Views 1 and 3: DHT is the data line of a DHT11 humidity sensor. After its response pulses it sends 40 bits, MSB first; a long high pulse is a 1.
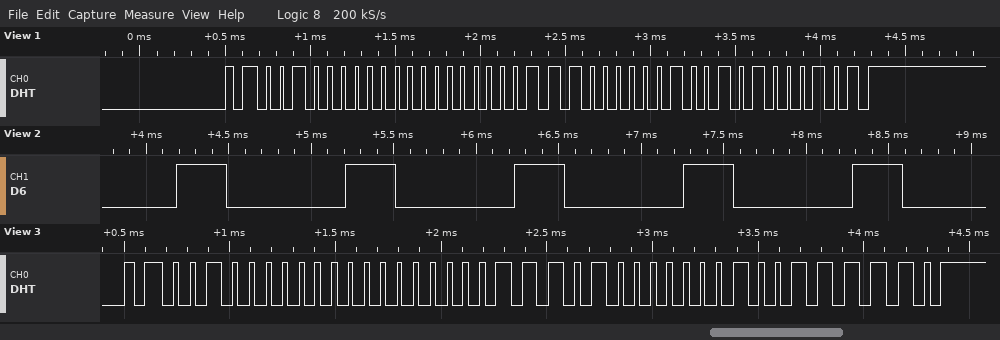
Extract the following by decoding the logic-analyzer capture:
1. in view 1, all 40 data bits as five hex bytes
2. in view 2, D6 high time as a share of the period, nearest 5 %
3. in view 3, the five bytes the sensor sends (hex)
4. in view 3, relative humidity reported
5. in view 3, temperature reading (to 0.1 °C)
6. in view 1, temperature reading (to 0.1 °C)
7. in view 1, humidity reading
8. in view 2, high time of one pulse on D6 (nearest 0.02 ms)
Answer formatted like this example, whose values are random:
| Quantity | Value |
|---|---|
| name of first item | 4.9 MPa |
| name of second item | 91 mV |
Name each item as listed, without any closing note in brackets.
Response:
| Quantity | Value |
|---|---|
| in view 1, all 40 data bits as five hex bytes | 20 00 1C 09 45 |
| in view 2, D6 high time as a share of the period, nearest 5 % | 30 % |
| in view 3, the five bytes the sensor sends | 20 00 1D 01 3E |
| in view 3, relative humidity reported | 32 % |
| in view 3, temperature reading | 29.1 °C |
| in view 1, temperature reading | 28.9 °C |
| in view 1, humidity reading | 32 % |
| in view 2, high time of one pulse on D6 | 0.30 ms |
